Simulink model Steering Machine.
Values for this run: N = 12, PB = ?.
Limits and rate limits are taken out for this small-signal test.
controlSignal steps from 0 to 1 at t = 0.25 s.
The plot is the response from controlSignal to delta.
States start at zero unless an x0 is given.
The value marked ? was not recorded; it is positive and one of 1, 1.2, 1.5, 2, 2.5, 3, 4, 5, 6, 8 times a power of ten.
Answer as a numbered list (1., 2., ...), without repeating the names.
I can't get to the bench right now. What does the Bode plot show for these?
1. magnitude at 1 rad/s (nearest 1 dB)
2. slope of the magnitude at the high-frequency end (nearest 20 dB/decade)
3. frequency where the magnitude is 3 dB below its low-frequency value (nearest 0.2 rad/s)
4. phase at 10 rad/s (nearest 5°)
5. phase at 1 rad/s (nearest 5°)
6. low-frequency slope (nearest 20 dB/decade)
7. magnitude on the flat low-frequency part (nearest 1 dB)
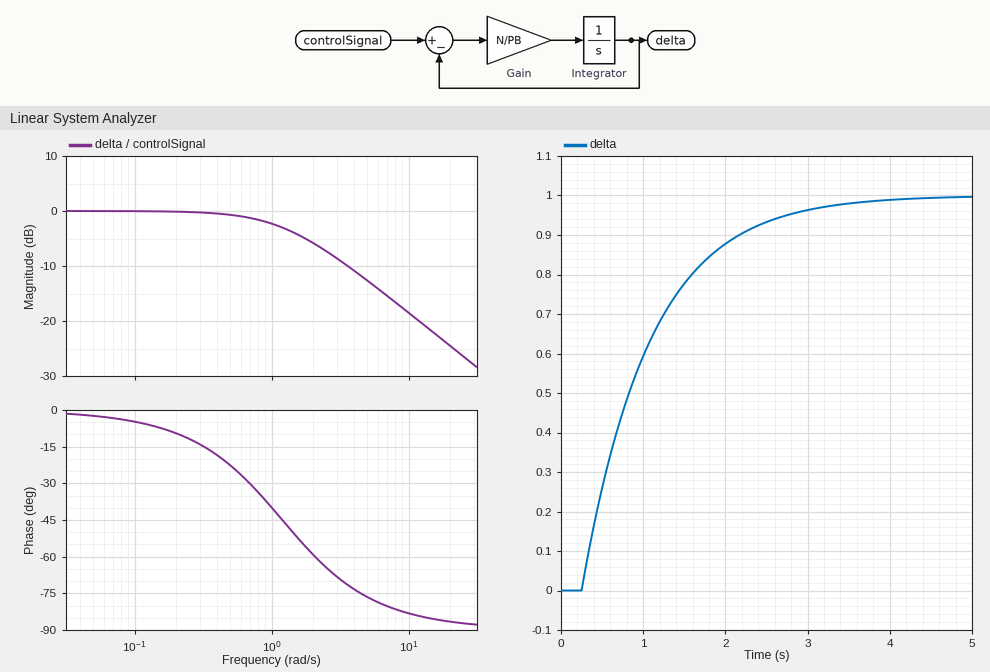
1. -2 dB
2. -20 dB/decade
3. 1.2 rad/s
4. -85°
5. -40°
6. 0 dB/decade
7. 0 dB
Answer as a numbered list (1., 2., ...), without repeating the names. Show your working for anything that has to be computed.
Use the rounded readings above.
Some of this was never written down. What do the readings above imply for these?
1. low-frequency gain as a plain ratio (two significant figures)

1. 10^(0 / 20) = 1.0
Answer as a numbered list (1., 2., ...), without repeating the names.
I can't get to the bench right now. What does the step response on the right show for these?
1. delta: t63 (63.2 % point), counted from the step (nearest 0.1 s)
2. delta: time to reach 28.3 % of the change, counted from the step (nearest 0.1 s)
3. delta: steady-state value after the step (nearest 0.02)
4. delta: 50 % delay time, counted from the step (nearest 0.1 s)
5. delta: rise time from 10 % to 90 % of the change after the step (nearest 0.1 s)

1. 0.8 s
2. 0.3 s
3. 1.00
4. 0.6 s
5. 1.8 s
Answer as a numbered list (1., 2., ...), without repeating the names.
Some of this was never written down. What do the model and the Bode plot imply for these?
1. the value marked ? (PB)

1. 10
